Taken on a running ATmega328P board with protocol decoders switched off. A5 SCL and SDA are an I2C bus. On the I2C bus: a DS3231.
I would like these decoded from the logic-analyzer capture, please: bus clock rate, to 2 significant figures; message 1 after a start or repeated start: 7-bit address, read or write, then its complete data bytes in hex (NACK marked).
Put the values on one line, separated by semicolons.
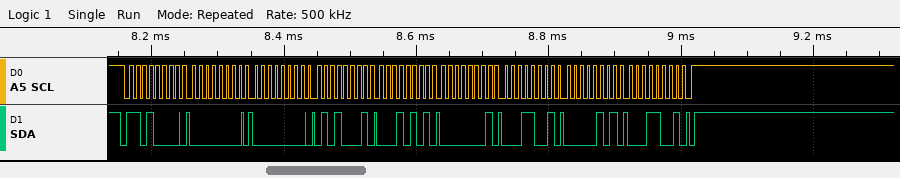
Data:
100 kHz; 0x68 write: 00 00 51 15 01 19 05 19
